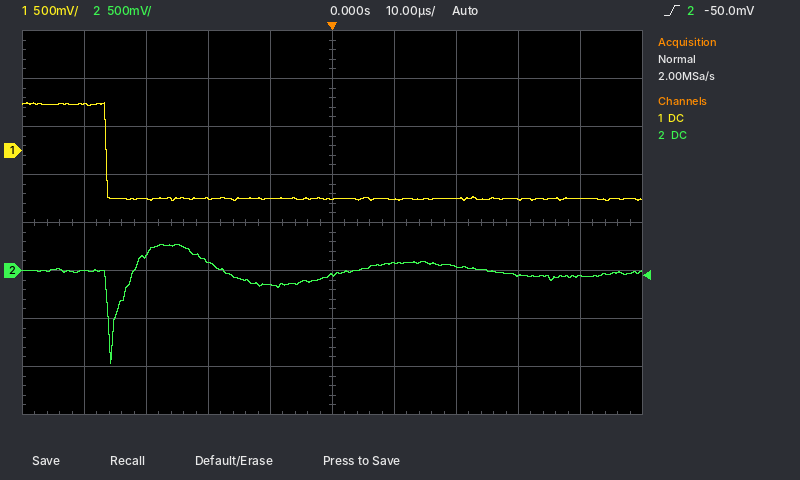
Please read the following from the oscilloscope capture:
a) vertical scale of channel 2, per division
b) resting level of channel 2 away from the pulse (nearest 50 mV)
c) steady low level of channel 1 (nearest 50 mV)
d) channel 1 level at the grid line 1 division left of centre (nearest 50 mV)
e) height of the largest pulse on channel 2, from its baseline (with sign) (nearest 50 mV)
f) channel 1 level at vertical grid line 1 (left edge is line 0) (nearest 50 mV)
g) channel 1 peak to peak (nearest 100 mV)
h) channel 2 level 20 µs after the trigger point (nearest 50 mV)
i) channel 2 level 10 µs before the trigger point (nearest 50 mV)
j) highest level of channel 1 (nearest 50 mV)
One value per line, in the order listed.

500 mV
0 mV
-500 mV
-500 mV
-950 mV
500 mV
1.00 V
50 mV
-150 mV
500 mV
